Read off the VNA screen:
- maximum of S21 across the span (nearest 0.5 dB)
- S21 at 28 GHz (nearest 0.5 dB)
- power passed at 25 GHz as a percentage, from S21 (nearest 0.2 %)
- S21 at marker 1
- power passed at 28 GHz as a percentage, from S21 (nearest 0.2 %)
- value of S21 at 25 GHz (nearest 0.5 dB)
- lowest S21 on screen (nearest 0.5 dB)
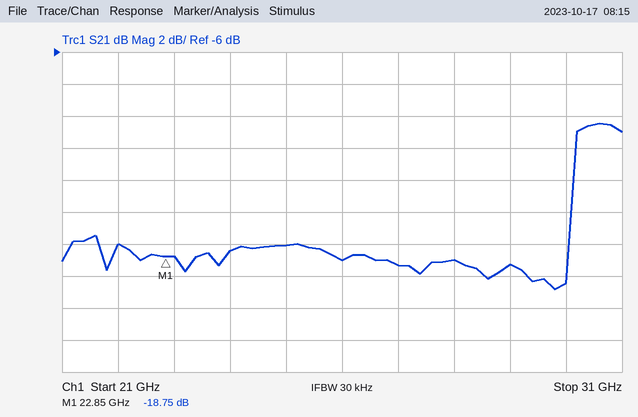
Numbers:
-10.5 dB
-19.0 dB
1.6 %
-18.75 dB
1.2 %
-18.0 dB
-21.0 dB
